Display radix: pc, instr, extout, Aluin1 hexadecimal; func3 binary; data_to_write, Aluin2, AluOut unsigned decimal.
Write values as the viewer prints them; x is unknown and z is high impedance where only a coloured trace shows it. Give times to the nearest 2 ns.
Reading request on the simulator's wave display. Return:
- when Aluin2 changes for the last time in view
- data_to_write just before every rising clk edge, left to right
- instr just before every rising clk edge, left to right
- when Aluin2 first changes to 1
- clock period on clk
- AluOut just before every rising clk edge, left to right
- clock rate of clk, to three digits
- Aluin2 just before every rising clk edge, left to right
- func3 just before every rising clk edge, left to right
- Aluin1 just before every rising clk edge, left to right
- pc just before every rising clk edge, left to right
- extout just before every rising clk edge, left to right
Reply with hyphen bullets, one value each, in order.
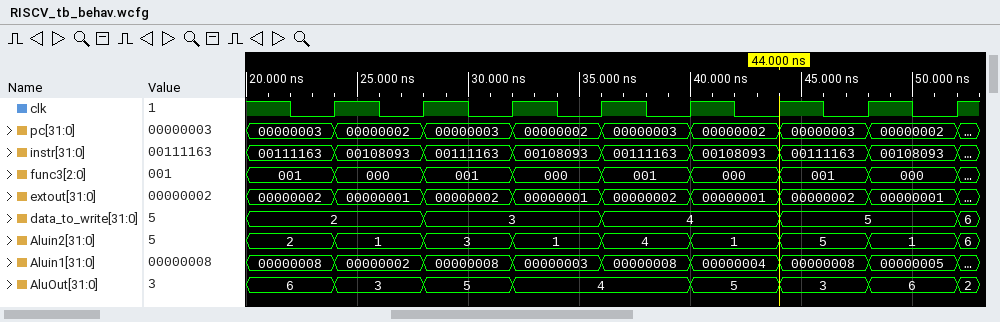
- 52 ns
- 2, 2, 3, 3, 4, 4, 5, 5
- 00111163, 00108093, 00111163, 00108093, 00111163, 00108093, 00111163, 00108093
- 24 ns
- 4 ns
- 6, 3, 5, 4, 4, 5, 3, 6
- 250 MHz
- 2, 1, 3, 1, 4, 1, 5, 1
- 001, 000, 001, 000, 001, 000, 001, 000
- 00000008, 00000002, 00000008, 00000003, 00000008, 00000004, 00000008, 00000005
- 00000003, 00000002, 00000003, 00000002, 00000003, 00000002, 00000003, 00000002
- 00000002, 00000001, 00000002, 00000001, 00000002, 00000001, 00000002, 00000001
